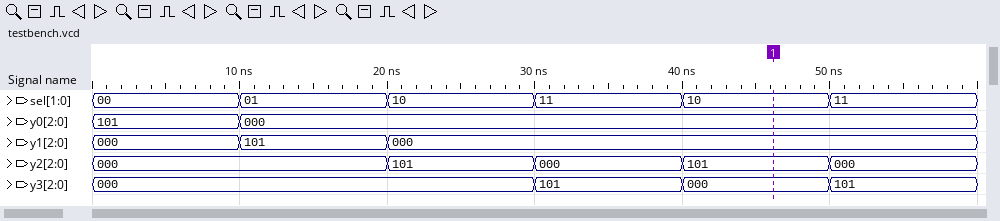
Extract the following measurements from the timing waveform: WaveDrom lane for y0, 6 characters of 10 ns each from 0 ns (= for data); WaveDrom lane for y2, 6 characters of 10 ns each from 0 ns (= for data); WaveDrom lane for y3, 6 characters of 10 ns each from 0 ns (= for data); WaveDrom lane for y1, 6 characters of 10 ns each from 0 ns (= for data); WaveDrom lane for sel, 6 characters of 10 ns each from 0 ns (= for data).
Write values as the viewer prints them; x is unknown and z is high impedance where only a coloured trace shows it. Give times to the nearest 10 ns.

{name: 'y0', wave: '==....', data: '101 000'}
{name: 'y2', wave: '=.====', data: '000 101 000 101 000'}
{name: 'y3', wave: '=..===', data: '000 101 000 101'}
{name: 'y1', wave: '===...', data: '000 101 000'}
{name: 'sel', wave: '======', data: '00 01 10 11 10 11'}
